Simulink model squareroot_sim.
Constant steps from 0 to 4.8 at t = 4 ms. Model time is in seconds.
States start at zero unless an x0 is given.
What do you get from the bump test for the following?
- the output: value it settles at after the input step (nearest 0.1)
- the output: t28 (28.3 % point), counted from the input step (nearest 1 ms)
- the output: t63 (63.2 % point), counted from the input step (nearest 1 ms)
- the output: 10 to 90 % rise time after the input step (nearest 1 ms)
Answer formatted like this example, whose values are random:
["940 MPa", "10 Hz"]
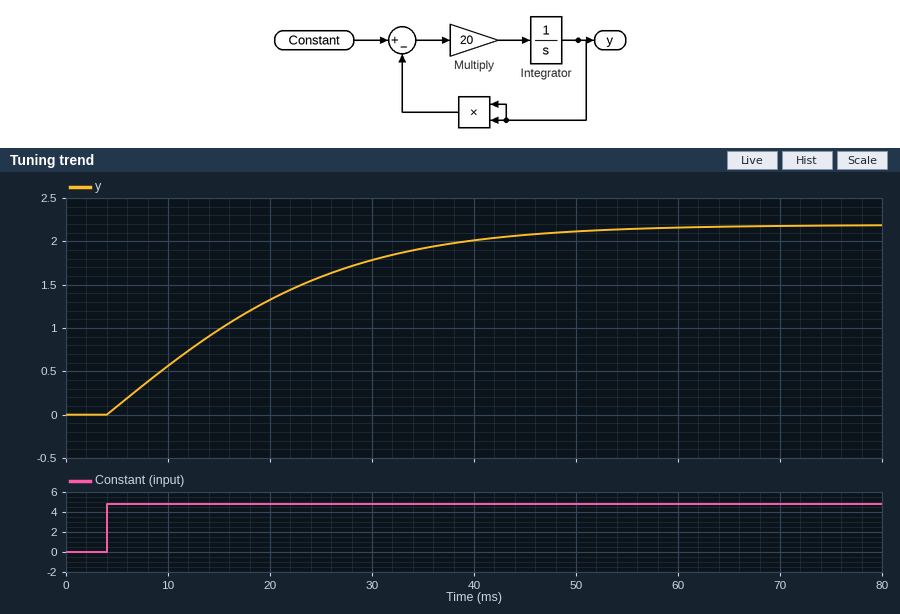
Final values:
["2.2", "7 ms", "17 ms", "31 ms"]
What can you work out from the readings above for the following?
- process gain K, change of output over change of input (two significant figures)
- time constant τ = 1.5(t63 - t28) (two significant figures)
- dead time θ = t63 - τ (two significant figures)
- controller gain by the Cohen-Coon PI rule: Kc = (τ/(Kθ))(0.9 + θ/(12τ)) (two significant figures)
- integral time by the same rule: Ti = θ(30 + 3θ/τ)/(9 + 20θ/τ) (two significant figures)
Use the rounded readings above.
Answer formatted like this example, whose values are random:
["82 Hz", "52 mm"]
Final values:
["0.46", "15 ms", "2.0 ms", "15", "5.2 ms"]
